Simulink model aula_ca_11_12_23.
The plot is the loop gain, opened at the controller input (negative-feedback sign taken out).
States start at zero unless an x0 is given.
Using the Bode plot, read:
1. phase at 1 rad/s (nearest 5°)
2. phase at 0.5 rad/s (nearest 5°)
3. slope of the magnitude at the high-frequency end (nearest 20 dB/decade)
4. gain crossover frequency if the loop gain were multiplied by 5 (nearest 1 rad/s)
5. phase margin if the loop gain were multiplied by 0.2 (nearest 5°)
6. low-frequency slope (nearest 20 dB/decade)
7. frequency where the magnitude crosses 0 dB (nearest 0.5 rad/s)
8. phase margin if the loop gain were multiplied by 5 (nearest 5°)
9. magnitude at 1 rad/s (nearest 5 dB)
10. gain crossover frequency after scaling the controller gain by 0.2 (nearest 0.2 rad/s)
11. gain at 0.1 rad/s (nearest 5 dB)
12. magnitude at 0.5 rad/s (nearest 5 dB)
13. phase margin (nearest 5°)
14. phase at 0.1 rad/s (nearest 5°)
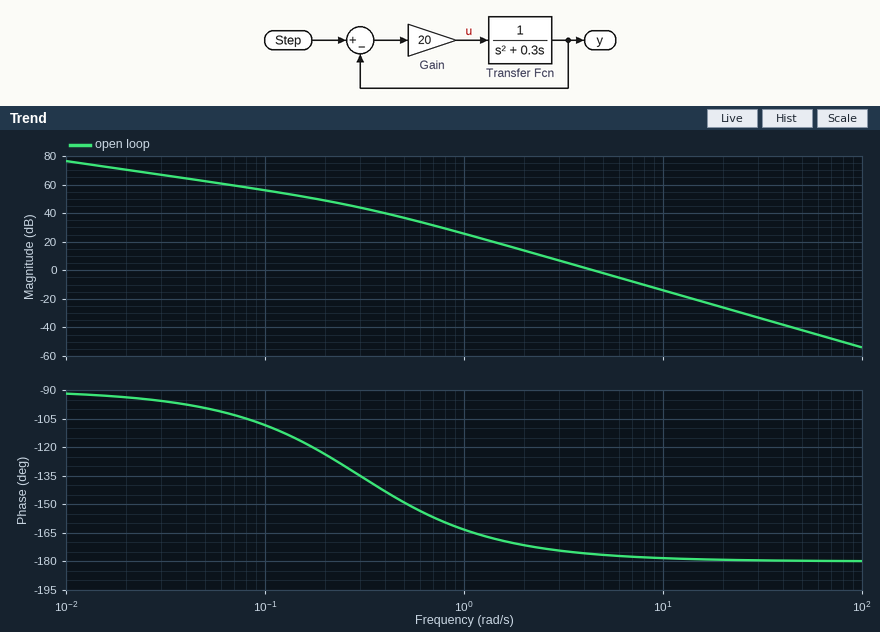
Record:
-165°
-150°
-40 dB/decade
10 rad/s
10°
-20 dB/decade
4.5 rad/s
0°
25 dB
2.0 rad/s
55 dB
35 dB
5°
-110°
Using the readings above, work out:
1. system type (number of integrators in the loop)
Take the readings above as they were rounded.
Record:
1
